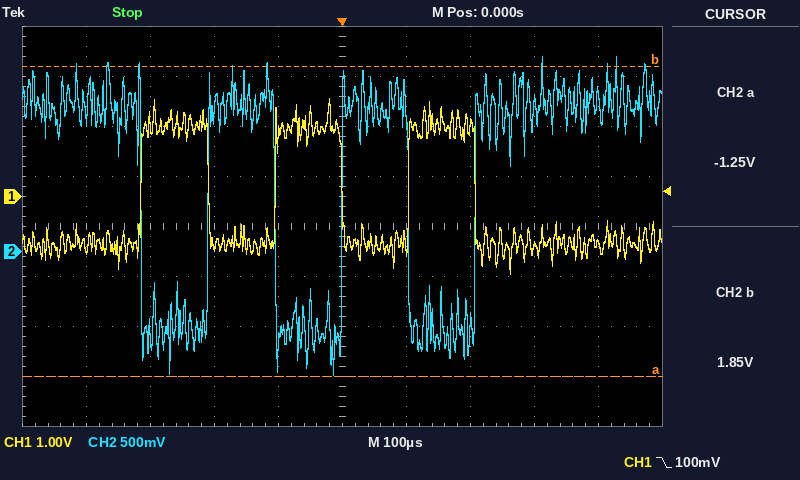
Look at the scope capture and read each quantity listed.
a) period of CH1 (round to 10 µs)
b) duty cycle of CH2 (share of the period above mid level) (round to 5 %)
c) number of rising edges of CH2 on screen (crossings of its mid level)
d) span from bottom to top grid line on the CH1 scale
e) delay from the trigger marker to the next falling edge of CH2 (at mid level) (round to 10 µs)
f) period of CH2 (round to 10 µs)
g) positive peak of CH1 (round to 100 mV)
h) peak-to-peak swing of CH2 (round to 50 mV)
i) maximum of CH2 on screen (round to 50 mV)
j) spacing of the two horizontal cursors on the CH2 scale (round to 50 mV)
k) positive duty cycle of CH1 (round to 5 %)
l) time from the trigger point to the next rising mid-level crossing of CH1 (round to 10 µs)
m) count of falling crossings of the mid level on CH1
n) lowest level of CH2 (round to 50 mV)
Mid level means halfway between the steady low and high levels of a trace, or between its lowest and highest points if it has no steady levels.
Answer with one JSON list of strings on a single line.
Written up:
["210 µs", "50 %", "3", "8 V", "100 µs", "210 µs", "2.0 V", "3.20 V", "1.95 V", "3.10 V", "50 %", "100 µs", "3", "-1.25 V"]
